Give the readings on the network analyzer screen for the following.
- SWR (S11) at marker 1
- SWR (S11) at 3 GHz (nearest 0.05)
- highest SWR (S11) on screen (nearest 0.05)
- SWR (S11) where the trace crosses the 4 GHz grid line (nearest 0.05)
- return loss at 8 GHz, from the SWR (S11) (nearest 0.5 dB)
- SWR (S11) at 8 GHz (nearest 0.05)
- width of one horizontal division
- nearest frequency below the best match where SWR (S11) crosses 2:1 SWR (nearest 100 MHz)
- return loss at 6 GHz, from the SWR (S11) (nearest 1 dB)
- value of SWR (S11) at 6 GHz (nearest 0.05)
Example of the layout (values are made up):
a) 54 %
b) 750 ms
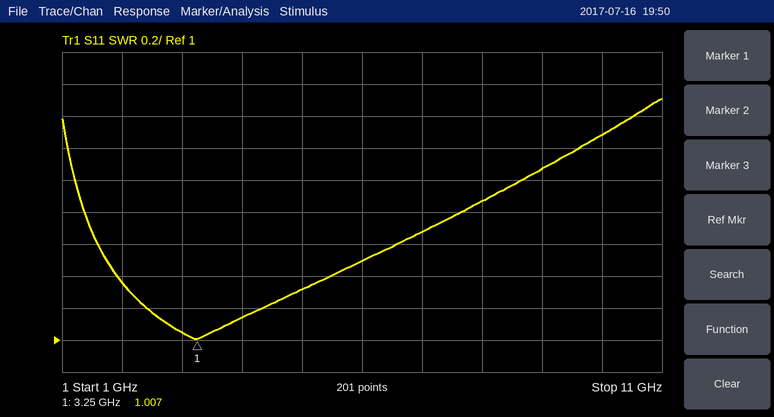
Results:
a) 1.007
b) 1.05
c) 2.50
d) 1.15
e) 10.5 dB
f) 1.85
g) 1 GHz
h) 1.2 GHz
i) 14 dB
j) 1.50
